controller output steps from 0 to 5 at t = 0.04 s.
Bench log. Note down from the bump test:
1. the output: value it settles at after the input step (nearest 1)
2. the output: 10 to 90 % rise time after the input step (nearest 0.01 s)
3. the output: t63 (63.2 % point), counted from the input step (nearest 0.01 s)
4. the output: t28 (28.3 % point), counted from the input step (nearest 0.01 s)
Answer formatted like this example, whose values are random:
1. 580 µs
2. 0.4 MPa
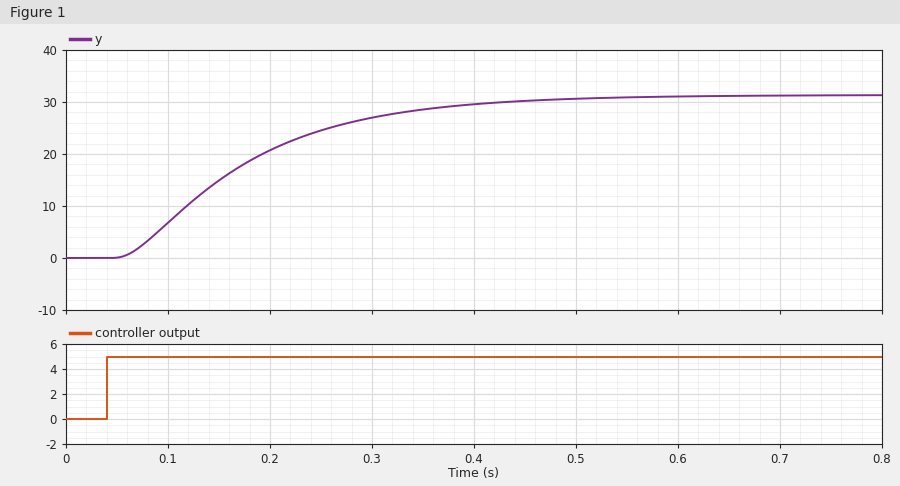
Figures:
1. 31
2. 0.26 s
3. 0.15 s
4. 0.07 s
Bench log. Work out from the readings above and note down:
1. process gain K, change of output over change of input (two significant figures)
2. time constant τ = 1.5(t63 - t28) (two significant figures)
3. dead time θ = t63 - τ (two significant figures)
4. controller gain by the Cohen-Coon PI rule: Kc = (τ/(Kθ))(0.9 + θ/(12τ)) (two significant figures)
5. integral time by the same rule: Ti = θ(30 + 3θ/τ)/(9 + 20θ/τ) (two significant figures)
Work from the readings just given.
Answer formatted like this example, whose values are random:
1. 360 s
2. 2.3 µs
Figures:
1. 6.2
2. 0.12 s
3. 0.030 s
4. 0.59
5. 0.066 s
